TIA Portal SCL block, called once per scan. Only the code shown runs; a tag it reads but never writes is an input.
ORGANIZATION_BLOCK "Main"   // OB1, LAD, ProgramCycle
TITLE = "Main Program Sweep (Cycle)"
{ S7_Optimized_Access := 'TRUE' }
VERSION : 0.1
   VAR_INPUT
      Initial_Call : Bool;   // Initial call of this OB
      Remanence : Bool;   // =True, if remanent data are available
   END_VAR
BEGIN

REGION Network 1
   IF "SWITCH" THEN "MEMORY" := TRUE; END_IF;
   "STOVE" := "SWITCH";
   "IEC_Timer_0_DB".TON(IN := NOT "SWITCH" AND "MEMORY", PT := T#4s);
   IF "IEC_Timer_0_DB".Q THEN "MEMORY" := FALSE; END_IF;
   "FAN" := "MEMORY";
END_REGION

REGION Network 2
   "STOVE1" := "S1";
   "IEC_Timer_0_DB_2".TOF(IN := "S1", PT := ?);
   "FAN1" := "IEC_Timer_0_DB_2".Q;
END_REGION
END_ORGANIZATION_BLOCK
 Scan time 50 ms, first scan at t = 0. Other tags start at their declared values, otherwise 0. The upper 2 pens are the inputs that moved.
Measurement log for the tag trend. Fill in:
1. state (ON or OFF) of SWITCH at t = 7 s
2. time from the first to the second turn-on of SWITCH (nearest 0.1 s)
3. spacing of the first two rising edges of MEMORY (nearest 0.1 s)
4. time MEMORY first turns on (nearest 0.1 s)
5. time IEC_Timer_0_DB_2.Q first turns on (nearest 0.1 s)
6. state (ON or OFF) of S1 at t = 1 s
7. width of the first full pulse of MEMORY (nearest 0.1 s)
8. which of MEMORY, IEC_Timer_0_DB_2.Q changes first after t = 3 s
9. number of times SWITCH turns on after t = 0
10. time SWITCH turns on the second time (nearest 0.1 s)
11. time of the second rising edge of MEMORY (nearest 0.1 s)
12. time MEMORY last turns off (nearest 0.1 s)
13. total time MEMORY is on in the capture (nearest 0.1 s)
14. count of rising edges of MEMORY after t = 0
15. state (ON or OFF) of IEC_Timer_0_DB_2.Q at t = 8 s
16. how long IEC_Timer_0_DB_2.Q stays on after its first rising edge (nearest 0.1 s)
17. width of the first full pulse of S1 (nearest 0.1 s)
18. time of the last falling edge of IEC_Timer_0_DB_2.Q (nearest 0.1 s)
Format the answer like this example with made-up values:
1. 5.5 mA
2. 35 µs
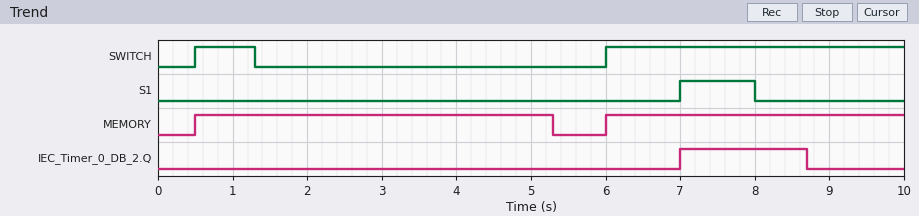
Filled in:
1. ON
2. 5.5 s
3. 5.5 s
4. 0.5 s
5. 7.0 s
6. OFF
7. 4.8 s
8. MEMORY
9. 2
10. 6.0 s
11. 6.0 s
12. 5.3 s
13. 8.8 s
14. 2
15. ON
16. 1.7 s
17. 1.0 s
18. 8.7 s
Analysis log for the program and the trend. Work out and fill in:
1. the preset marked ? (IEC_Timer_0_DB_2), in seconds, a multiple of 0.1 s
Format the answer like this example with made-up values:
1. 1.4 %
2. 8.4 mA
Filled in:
1. 0.7 s
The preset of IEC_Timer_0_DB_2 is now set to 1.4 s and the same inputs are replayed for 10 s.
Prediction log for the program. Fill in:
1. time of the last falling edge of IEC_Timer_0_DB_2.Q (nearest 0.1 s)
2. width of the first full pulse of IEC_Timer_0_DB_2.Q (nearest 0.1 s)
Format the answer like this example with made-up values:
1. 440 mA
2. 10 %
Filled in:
1. 9.4 s
2. 2.4 s
